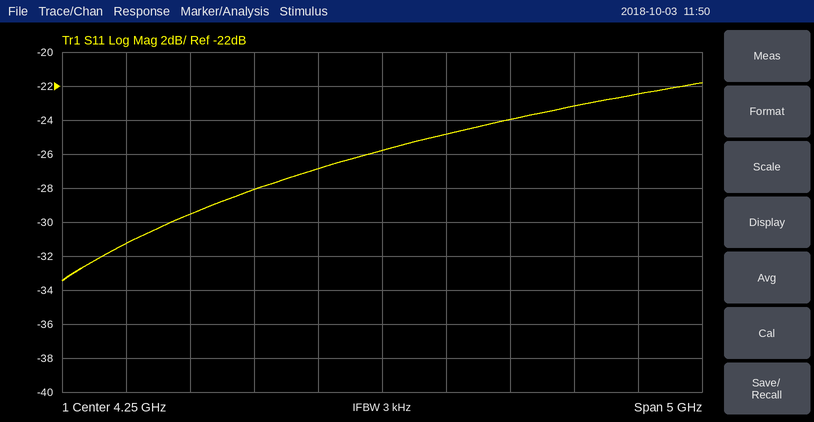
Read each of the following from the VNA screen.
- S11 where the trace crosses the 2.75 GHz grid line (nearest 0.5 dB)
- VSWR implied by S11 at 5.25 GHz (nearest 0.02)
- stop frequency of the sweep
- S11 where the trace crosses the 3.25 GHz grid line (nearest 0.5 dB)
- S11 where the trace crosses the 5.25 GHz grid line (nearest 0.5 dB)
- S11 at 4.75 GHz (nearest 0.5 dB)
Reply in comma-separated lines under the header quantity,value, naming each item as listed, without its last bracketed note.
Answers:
quantity,value
S11 where the trace crosses the 2.75 GHz grid line,-29.5 dB
VSWR implied by S11 at 5.25 GHz,1.14
stop frequency of the sweep,6.75 GHz
S11 where the trace crosses the 3.25 GHz grid line,-28.0 dB
S11 where the trace crosses the 5.25 GHz grid line,-24.0 dB
S11 at 4.75 GHz,-25.0 dB
